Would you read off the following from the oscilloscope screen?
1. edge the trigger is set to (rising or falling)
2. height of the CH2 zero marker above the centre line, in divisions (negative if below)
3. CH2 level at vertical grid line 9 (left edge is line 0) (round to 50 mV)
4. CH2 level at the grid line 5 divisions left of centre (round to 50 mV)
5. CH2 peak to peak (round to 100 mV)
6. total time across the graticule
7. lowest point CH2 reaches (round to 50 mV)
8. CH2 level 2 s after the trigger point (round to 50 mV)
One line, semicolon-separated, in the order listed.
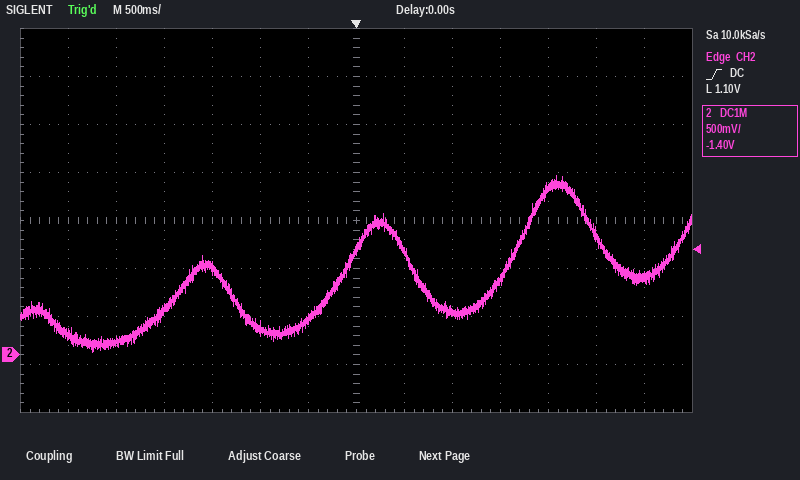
rising; -2.8 div; 450 mV; 150 mV; 1.80 V; 7 s; 50 mV; 1.75 V
